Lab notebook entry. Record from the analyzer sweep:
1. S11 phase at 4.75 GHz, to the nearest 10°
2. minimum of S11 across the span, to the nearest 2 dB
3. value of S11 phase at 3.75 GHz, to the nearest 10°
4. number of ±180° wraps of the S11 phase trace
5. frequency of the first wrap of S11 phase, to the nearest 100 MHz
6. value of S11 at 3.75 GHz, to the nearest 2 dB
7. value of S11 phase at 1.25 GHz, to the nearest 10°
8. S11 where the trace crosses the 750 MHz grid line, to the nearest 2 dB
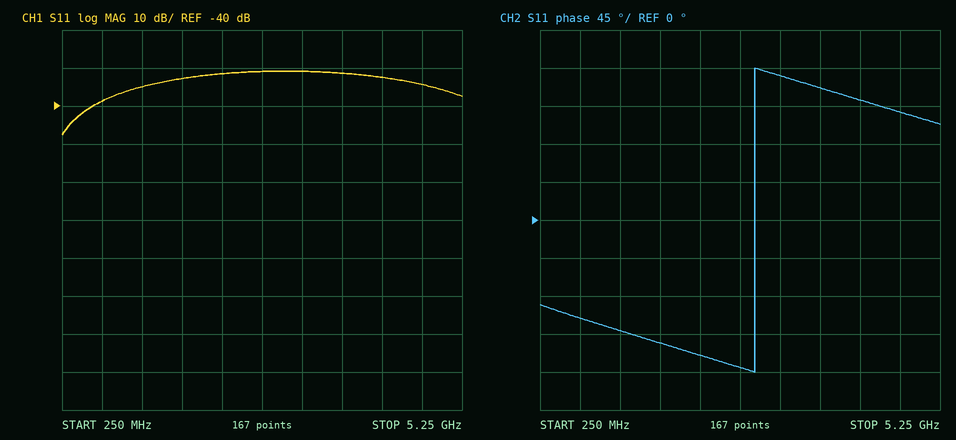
130°
-48 dB
160°
1
2.9 GHz
-32 dB
-130°
-38 dB
